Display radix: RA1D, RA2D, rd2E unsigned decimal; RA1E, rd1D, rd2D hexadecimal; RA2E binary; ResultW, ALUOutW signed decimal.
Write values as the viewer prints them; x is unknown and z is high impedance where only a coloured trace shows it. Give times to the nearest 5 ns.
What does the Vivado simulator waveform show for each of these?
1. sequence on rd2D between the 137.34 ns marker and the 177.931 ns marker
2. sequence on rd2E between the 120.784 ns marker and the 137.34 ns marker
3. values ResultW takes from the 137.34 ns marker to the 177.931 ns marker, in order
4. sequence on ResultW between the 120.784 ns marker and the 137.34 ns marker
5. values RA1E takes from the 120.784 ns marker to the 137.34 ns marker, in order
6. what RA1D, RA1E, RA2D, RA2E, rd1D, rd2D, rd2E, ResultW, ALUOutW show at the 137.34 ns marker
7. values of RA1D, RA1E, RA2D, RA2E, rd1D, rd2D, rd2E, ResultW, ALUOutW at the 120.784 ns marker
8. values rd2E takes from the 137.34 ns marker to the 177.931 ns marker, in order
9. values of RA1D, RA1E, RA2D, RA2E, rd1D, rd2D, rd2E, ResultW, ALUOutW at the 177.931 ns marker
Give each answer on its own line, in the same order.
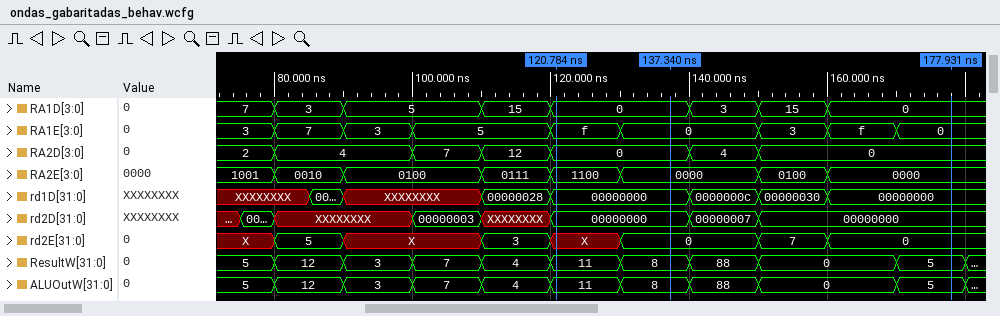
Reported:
00000000, 00000007, 00000000
X, 0
8, 88, 0, 5
11, 8
f, 0
RA1D=0, RA1E=0, RA2D=0, RA2E=0000, rd1D=00000000, rd2D=00000000, rd2E=0, ResultW=8, ALUOutW=8
RA1D=0, RA1E=f, RA2D=0, RA2E=1100, rd1D=00000000, rd2D=00000000, rd2E=X, ResultW=11, ALUOutW=11
0, 7, 0
RA1D=0, RA1E=0, RA2D=0, RA2E=0000, rd1D=00000000, rd2D=00000000, rd2E=0, ResultW=5, ALUOutW=5
